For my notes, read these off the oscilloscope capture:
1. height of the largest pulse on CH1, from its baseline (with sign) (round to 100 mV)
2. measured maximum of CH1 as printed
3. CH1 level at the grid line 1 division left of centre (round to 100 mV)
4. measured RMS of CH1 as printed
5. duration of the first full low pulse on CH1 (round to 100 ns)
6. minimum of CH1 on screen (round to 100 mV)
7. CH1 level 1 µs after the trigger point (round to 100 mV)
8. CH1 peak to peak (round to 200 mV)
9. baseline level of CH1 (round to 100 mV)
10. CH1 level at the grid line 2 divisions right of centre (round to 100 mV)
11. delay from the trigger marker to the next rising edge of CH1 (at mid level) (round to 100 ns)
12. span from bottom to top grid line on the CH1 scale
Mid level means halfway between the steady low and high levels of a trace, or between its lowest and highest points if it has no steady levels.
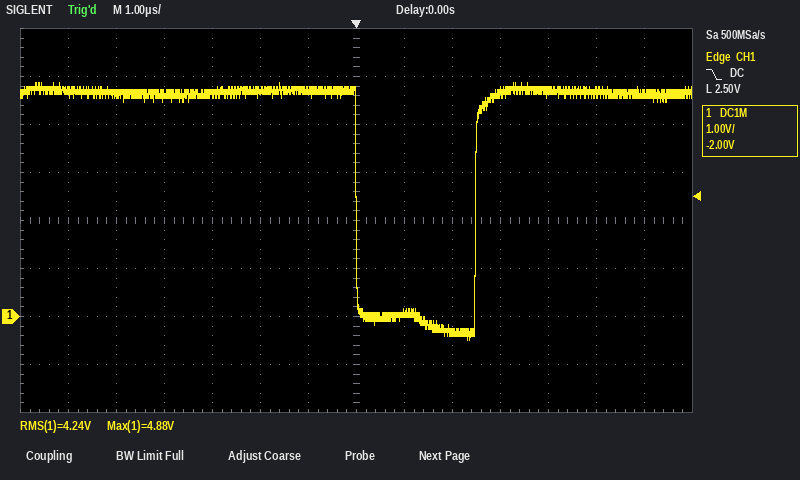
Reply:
-5.2 V
4.88 V
4.7 V
4.24 V
2.5 µs
-500 mV
100 mV
5.4 V
4.7 V
-300 mV
2.5 µs
8 V
